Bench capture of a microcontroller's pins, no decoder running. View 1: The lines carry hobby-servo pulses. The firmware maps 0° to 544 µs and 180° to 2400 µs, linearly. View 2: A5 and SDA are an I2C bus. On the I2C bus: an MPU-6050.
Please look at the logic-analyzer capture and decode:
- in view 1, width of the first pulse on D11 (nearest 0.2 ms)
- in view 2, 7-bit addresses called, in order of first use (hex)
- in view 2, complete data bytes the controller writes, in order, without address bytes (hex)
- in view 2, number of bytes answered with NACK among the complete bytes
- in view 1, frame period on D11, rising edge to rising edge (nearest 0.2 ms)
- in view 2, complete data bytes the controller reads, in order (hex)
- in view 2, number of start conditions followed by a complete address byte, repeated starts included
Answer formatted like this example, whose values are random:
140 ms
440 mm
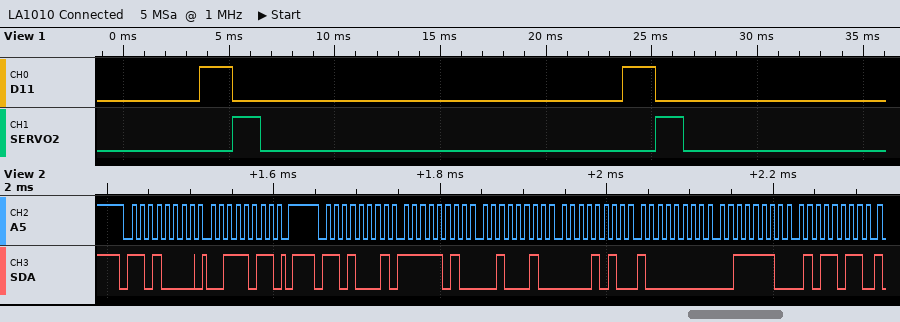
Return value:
1.6 ms
0x68
3B
0
20.0 ms
FA 22 0A 80 3E 5B
2
